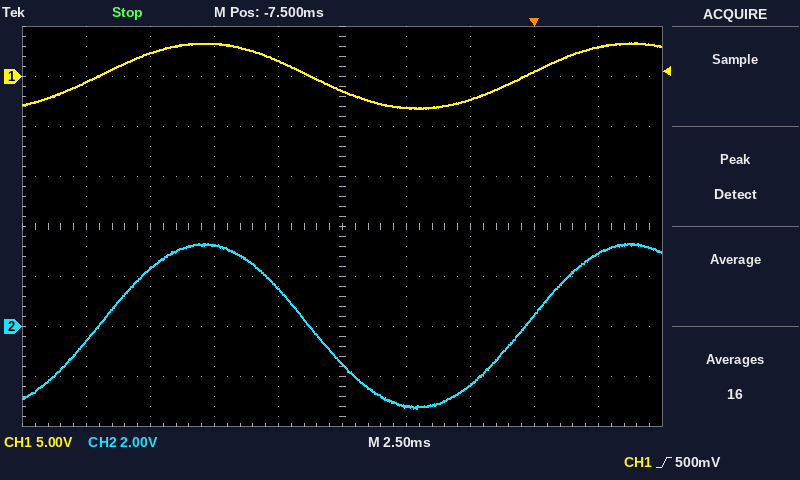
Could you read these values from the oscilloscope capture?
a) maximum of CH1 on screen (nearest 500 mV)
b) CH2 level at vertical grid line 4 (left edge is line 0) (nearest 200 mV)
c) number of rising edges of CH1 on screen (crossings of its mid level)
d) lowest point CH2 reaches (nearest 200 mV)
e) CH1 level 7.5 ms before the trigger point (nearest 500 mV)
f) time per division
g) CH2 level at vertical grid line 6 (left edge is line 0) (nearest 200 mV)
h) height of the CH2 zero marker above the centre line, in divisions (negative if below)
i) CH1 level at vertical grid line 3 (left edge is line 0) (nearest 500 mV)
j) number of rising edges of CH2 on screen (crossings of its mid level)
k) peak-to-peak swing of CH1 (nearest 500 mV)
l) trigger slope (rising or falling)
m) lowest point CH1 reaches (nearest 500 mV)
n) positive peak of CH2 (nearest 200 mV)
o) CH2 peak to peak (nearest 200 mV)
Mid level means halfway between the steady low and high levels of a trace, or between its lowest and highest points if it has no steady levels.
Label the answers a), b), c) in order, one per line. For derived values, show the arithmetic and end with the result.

a) 3.5 V
b) 1.6 V
c) 2
d) -3.2 V
e) -1.5 V
f) 2.5 ms
g) -3.2 V
h) -2.0 div
i) 3.5 V
j) 2
k) 3.5 V − (-3.0 V) = 6.5 V
l) rising
m) -3.0 V
n) 3.4 V
o) 3.4 V − (-3.2 V) = 6.6 V
